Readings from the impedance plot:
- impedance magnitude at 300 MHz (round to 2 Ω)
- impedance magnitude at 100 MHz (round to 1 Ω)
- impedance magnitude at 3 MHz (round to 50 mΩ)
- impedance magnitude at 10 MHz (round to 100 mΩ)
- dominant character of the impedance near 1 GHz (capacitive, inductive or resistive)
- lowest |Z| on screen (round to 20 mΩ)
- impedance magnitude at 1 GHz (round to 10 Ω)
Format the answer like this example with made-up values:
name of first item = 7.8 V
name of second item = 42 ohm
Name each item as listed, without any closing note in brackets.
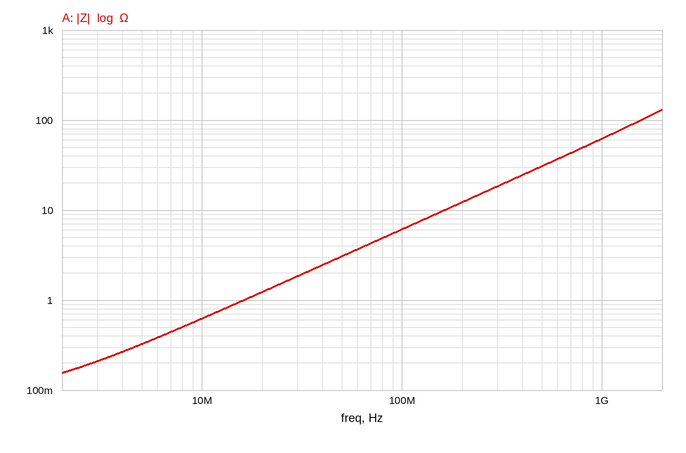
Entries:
impedance magnitude at 300 MHz = 18 Ω
impedance magnitude at 100 MHz = 6 Ω
impedance magnitude at 3 MHz = 200 mΩ
impedance magnitude at 10 MHz = 600 mΩ
dominant character of the impedance near 1 GHz = inductive
lowest |Z| on screen = 160 mΩ
impedance magnitude at 1 GHz = 60 Ω
